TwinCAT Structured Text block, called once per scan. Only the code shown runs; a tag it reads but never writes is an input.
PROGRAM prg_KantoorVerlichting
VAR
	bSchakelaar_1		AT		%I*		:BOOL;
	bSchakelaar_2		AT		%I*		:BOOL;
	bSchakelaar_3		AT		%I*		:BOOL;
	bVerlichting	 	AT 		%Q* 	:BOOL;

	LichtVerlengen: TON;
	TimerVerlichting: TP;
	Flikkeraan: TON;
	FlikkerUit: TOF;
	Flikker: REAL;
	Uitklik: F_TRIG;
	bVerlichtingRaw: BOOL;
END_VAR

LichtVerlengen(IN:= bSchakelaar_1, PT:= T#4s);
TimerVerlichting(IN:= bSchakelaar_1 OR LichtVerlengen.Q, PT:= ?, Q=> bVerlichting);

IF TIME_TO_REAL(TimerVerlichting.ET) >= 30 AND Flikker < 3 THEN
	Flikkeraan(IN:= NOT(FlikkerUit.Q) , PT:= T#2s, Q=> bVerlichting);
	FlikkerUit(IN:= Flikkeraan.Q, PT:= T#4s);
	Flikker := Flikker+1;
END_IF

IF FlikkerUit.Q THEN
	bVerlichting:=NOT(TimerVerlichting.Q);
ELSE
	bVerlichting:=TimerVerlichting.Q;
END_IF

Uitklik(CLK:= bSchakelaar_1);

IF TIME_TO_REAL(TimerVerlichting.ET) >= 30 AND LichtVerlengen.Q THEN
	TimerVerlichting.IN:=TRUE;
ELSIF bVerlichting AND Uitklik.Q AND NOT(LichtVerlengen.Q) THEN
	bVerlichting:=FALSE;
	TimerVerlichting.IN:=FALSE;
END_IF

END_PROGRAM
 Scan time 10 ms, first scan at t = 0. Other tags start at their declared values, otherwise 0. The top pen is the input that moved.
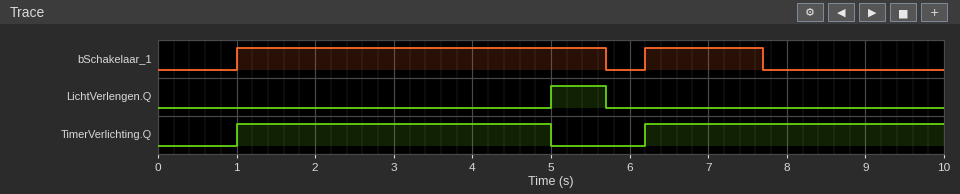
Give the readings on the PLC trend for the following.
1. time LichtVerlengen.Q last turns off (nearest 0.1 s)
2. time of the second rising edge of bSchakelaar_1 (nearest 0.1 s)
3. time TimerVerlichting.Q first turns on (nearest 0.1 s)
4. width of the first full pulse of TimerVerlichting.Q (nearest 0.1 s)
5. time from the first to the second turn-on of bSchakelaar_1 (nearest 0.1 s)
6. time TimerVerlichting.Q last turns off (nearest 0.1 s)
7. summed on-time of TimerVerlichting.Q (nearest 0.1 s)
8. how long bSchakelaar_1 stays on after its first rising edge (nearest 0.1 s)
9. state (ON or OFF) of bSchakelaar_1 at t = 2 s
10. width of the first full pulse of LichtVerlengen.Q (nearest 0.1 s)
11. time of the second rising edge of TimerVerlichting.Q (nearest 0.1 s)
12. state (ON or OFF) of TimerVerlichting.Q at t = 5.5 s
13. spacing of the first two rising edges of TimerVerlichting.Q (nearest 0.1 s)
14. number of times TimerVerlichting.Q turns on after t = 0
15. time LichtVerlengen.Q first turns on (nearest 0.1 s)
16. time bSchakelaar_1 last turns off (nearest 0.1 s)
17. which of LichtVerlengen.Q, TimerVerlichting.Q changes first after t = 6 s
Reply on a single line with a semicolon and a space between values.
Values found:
5.7 s; 6.2 s; 1.0 s; 4.0 s; 5.2 s; 5.0 s; 7.8 s; 4.7 s; ON; 0.7 s; 6.2 s; OFF; 5.2 s; 2; 5.0 s; 7.7 s; TimerVerlichting.Q
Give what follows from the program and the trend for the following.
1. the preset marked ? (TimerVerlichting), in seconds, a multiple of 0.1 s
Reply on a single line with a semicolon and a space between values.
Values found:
4.0 s
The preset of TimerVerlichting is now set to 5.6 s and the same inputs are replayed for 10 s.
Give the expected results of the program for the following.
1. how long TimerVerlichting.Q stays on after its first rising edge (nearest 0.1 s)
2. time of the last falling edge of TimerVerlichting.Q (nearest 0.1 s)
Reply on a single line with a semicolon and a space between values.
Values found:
5.6 s; 6.6 s
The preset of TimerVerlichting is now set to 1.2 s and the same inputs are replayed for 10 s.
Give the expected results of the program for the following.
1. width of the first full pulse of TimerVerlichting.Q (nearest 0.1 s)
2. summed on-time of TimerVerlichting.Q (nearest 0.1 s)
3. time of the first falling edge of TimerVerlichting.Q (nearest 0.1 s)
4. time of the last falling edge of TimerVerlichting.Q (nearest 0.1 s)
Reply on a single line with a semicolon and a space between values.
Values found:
1.2 s; 2.4 s; 2.2 s; 7.4 s
